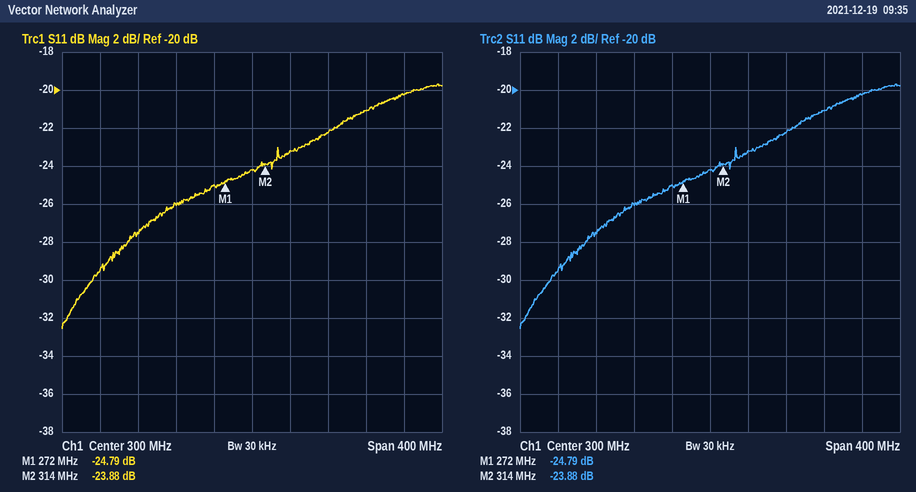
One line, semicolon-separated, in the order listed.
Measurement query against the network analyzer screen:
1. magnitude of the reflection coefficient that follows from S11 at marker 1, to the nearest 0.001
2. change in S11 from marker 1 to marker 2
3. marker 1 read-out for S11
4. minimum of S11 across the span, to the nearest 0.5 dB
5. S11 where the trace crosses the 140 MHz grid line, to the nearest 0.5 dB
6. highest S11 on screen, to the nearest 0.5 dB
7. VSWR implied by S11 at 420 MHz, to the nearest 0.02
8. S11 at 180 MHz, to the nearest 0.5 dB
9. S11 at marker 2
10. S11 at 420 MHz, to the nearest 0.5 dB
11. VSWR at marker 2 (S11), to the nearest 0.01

0.058; 0.91 dB; -24.79 dB; -32.5 dB; -29.5 dB; -19.5 dB; 1.20; -27.5 dB; -23.88 dB; -21.0 dB; 1.14
